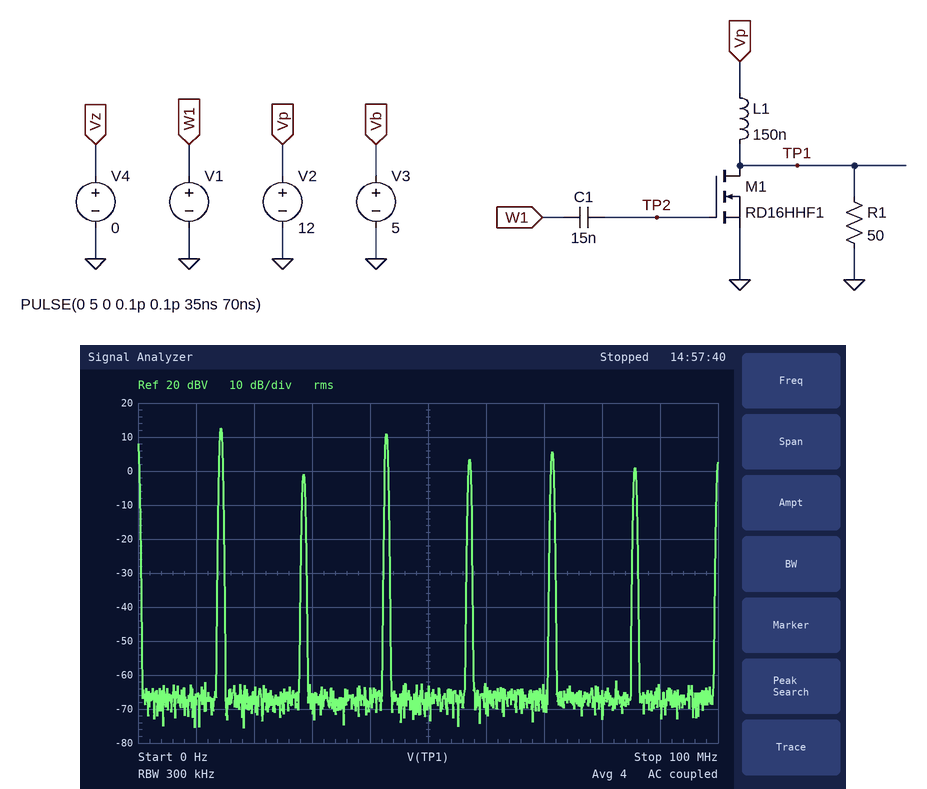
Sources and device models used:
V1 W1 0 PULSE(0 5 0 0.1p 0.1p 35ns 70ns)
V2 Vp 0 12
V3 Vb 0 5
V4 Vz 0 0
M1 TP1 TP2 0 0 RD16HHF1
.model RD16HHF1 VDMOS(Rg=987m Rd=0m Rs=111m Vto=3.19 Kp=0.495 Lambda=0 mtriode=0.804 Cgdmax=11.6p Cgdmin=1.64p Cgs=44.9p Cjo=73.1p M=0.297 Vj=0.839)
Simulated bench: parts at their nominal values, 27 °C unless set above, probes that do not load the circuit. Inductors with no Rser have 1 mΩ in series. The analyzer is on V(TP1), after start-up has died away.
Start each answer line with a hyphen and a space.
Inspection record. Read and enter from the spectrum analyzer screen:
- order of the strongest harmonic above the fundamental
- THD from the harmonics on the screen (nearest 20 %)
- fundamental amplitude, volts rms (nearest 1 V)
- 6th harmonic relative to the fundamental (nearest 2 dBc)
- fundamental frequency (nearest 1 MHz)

- 3
- 100 %
- 4 V
- -12 dBc
- 14 MHz
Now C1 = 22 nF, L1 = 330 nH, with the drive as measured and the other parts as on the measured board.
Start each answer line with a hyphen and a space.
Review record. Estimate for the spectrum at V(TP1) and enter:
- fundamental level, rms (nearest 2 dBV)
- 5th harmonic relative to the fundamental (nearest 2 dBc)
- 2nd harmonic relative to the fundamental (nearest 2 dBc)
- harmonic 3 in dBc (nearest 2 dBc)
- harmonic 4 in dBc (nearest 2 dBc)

- 18 dBV
- -12 dBc
- -10 dBc
- -8 dBc
- -16 dBc
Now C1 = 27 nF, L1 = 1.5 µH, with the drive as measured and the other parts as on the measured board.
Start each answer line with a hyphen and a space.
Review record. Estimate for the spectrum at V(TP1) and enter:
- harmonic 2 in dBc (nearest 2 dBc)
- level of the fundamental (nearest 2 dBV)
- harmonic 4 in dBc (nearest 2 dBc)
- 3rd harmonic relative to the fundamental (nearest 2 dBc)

- -18 dBc
- 20 dBV
- -24 dBc
- -10 dBc
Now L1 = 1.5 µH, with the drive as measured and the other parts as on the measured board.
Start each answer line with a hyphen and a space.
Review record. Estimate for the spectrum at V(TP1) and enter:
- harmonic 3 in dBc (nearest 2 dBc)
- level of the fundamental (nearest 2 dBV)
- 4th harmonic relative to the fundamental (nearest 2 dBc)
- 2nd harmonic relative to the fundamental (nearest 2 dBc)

- -10 dBc
- 20 dBV
- -24 dBc
- -18 dBc
